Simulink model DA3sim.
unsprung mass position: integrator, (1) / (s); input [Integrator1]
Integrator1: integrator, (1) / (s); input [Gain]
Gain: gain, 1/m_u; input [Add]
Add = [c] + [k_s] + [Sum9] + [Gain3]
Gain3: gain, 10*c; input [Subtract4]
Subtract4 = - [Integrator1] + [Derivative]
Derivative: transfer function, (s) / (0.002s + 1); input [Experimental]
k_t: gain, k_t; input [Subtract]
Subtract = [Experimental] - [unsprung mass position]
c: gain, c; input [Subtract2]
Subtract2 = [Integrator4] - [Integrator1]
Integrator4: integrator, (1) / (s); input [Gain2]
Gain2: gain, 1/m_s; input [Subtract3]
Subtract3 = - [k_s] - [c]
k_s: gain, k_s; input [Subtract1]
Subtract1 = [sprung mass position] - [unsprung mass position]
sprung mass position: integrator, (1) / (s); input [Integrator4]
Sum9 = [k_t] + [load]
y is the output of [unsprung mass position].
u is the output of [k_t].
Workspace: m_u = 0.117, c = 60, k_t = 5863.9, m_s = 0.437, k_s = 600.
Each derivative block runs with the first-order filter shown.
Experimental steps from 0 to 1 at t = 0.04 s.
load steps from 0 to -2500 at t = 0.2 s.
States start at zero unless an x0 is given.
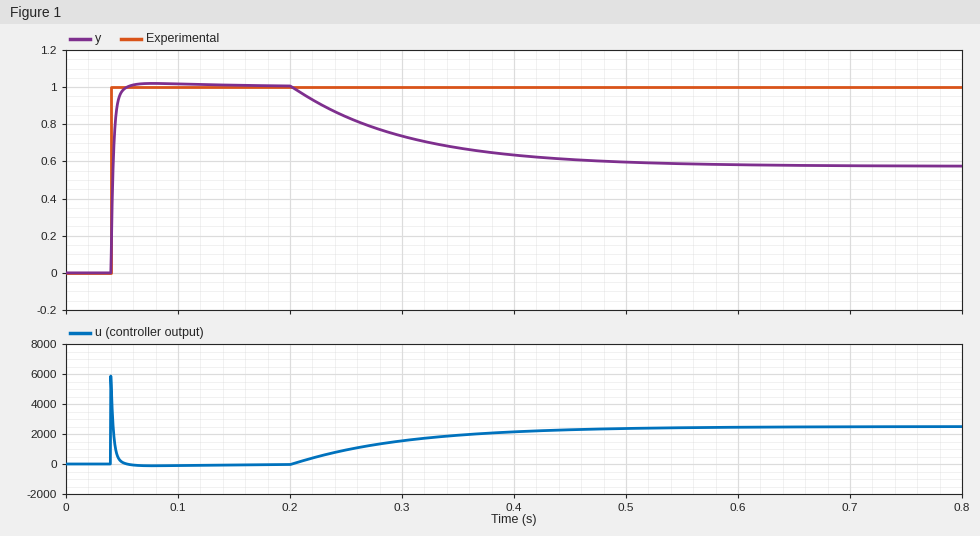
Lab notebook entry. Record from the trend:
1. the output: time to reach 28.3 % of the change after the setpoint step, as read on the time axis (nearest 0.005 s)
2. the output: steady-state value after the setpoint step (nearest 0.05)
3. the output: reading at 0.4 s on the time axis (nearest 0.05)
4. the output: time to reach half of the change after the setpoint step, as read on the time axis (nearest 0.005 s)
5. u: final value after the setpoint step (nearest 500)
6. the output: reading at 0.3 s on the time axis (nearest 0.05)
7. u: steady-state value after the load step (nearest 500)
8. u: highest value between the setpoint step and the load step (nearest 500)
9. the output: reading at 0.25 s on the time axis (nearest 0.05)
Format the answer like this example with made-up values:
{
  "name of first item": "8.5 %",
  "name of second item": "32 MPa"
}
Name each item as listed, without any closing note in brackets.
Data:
{
  "the output: time to reach 28.3 % of the change after the setpoint step, as read on the time axis": "0.040 s",
  "the output: steady-state value after the setpoint step": "1.00",
  "the output: reading at 0.4 s on the time axis": "0.65",
  "the output: time to reach half of the change after the setpoint step, as read on the time axis": "0.040 s",
  "u: final value after the setpoint step": "0",
  "the output: reading at 0.3 s on the time axis": "0.75",
  "u: steady-state value after the load step": "2500",
  "u: highest value between the setpoint step and the load step": "6000",
  "the output: reading at 0.25 s on the time axis": "0.85"
}
